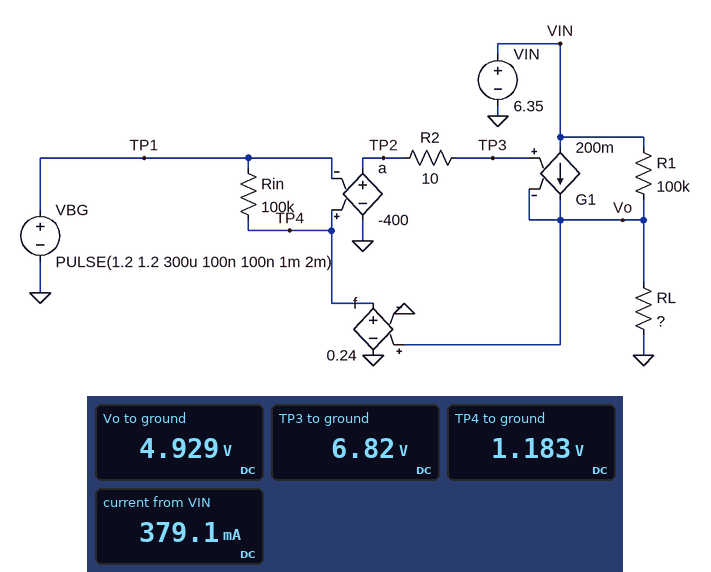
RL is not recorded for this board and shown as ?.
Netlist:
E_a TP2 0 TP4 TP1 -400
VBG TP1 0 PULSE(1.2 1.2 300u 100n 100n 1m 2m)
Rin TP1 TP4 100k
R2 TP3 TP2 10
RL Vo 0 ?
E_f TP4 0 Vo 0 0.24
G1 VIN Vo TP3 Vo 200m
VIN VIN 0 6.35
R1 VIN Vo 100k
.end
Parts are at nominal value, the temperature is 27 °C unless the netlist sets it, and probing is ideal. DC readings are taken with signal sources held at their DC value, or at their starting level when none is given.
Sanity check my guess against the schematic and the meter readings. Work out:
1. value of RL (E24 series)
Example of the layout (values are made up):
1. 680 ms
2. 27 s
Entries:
1. 13 Ω
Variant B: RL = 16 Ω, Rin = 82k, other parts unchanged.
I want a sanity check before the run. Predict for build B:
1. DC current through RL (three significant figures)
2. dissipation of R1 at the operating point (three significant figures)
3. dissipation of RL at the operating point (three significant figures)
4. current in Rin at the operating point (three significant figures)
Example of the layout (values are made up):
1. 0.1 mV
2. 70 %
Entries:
1. 308 mA
2. 20.1 µW
3. 1.52 W
4. 197 nA
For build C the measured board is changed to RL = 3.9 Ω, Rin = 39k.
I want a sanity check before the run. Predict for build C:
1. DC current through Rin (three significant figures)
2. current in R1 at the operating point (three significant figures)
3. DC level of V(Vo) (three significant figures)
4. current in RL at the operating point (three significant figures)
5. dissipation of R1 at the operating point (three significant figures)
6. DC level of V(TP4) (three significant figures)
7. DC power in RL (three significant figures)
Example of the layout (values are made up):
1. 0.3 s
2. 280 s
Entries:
1. 714 nA
2. 14.7 µA
3. 4.88 V
4. 1.25 A
5. 21.5 µW
6. 1.17 V
7. 6.12 W
